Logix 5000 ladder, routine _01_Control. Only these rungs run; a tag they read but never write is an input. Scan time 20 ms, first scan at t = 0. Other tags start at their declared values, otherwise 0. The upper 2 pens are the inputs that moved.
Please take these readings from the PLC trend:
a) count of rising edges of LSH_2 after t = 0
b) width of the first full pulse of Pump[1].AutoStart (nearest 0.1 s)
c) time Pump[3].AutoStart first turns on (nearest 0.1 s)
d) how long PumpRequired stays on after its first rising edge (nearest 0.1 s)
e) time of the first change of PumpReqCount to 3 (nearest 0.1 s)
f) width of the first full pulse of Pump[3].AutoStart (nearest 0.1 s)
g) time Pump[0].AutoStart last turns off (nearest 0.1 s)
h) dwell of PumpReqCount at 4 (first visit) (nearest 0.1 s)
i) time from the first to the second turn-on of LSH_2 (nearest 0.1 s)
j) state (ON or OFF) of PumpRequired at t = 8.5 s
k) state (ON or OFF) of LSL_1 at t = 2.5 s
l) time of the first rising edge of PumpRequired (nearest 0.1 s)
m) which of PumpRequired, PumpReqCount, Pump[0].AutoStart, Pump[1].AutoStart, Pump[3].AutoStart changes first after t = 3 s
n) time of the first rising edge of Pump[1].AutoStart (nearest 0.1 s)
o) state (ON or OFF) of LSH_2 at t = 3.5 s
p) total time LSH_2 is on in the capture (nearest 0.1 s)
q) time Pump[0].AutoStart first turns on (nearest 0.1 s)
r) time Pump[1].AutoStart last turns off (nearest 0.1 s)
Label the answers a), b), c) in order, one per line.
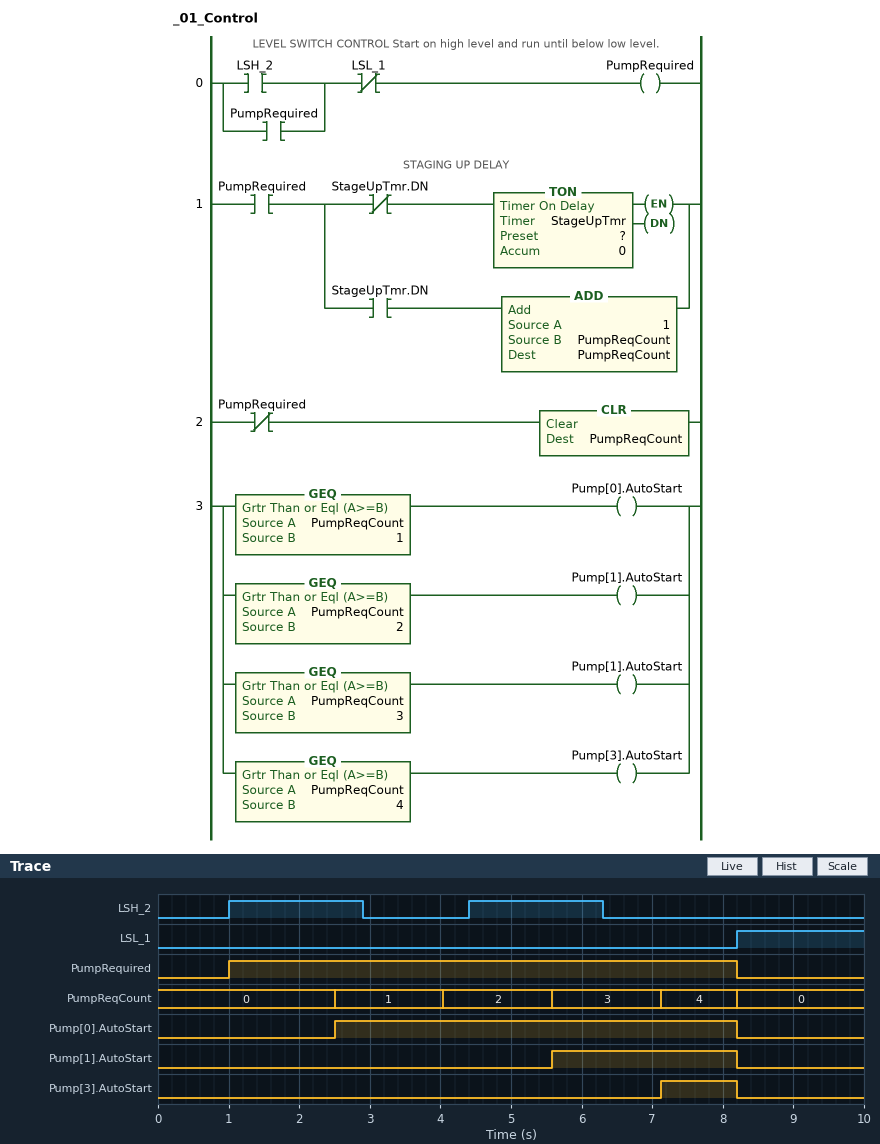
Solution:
a) 2
b) 2.6 s
c) 7.1 s
d) 7.2 s
e) 5.6 s
f) 1.1 s
g) 8.2 s
h) 1.1 s
i) 3.4 s
j) OFF
k) OFF
l) 1.0 s
m) PumpReqCount
n) 5.6 s
o) OFF
p) 3.8 s
q) 2.5 s
r) 8.2 s
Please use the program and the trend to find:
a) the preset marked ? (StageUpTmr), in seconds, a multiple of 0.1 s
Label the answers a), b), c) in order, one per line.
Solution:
a) 1.5 s
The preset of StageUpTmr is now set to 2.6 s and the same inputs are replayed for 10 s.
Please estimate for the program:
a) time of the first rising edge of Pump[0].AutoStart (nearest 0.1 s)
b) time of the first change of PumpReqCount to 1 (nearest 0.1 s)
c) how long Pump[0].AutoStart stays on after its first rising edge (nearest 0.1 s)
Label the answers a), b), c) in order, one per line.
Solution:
a) 3.6 s
b) 3.6 s
c) 4.6 s
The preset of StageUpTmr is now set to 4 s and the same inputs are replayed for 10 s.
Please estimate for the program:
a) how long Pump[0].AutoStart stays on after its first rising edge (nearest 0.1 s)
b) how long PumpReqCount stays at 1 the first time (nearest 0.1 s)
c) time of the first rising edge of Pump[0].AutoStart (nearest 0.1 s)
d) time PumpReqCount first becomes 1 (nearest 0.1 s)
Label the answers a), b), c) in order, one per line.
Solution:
a) 3.2 s
b) 3.2 s
c) 5.0 s
d) 5.0 s
